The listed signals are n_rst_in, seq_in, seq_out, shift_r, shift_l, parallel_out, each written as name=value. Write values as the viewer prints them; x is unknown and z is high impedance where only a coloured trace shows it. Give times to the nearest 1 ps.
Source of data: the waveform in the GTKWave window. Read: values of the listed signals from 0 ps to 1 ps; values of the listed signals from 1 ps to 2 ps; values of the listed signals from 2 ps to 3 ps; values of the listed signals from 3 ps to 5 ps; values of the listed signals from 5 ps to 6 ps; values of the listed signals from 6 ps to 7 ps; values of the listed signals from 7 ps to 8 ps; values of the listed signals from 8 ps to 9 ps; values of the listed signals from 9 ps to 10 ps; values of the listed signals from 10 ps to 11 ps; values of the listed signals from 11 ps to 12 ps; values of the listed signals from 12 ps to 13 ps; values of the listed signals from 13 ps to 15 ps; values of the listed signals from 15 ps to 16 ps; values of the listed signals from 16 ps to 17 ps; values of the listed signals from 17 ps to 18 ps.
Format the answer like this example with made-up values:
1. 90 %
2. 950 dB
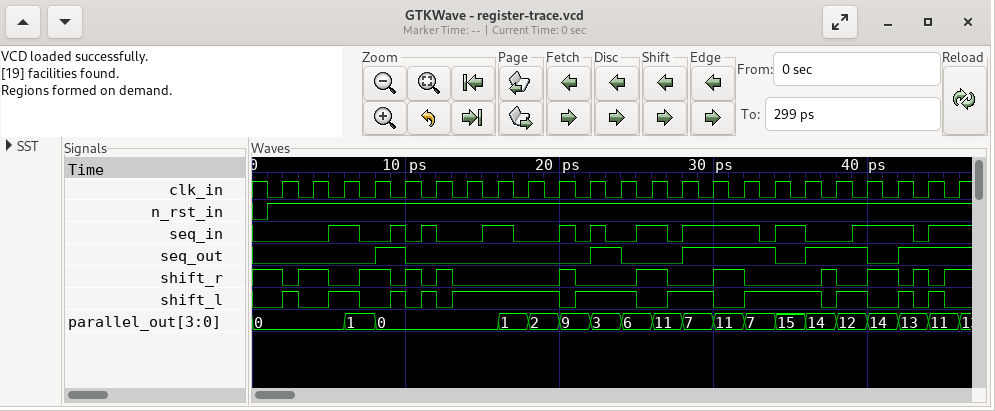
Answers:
1. n_rst_in=0, seq_in=0, seq_out=0, shift_r=1, shift_l=0, parallel_out=0
2. n_rst_in=1, seq_in=0, seq_out=0, shift_r=1, shift_l=0, parallel_out=0
3. n_rst_in=1, seq_in=0, seq_out=0, shift_r=0, shift_l=1, parallel_out=0
4. n_rst_in=1, seq_in=0, seq_out=0, shift_r=1, shift_l=0, parallel_out=0
5. n_rst_in=1, seq_in=1, seq_out=0, shift_r=0, shift_l=1, parallel_out=0
6. n_rst_in=1, seq_in=1, seq_out=0, shift_r=0, shift_l=1, parallel_out=1
7. n_rst_in=1, seq_in=0, seq_out=0, shift_r=1, shift_l=0, parallel_out=1
8. n_rst_in=1, seq_in=0, seq_out=1, shift_r=1, shift_l=0, parallel_out=0
9. n_rst_in=1, seq_in=1, seq_out=1, shift_r=0, shift_l=1, parallel_out=0
10. n_rst_in=1, seq_in=0, seq_out=0, shift_r=1, shift_l=0, parallel_out=0
11. n_rst_in=1, seq_in=1, seq_out=0, shift_r=0, shift_l=1, parallel_out=0
12. n_rst_in=1, seq_in=0, seq_out=0, shift_r=1, shift_l=0, parallel_out=0
13. n_rst_in=1, seq_in=0, seq_out=0, shift_r=0, shift_l=1, parallel_out=0
14. n_rst_in=1, seq_in=1, seq_out=0, shift_r=0, shift_l=1, parallel_out=0
15. n_rst_in=1, seq_in=1, seq_out=0, shift_r=0, shift_l=1, parallel_out=1
16. n_rst_in=1, seq_in=0, seq_out=0, shift_r=0, shift_l=1, parallel_out=1
